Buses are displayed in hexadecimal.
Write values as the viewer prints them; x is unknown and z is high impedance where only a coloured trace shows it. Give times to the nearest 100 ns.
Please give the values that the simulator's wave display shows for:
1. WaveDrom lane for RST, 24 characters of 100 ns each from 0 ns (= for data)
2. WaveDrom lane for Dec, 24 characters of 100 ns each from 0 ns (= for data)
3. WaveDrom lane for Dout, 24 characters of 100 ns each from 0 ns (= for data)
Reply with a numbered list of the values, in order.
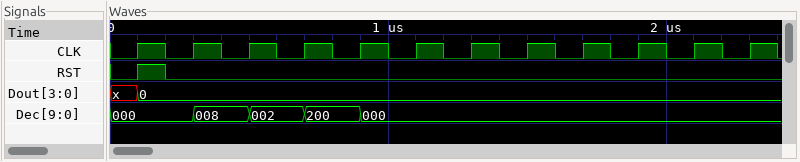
1. {name: 'RST', wave: '010.....................'}
2. {name: 'Dec', wave: '=..=.=.=.=..............', data: '000 008 002 200 000'}
3. {name: 'Dout', wave: 'x=......................', data: '0'}
